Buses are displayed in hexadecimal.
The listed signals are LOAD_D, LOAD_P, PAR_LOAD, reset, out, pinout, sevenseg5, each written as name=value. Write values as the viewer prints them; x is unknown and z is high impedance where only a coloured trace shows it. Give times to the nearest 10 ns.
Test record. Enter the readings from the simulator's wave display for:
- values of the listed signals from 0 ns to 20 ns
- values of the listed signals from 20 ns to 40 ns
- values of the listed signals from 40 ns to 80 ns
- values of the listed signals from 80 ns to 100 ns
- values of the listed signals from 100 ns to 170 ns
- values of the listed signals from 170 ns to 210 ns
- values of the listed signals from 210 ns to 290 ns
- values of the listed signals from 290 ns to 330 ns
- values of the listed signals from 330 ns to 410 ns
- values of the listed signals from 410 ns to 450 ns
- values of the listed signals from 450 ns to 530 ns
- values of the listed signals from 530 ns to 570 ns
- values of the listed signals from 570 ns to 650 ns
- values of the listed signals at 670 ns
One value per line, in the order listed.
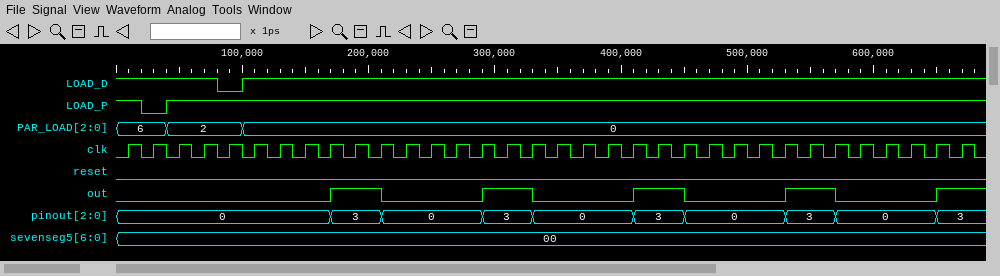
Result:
LOAD_D=1, LOAD_P=1, PAR_LOAD=6, reset=0, out=0, pinout=0, sevenseg5=00
LOAD_D=1, LOAD_P=0, PAR_LOAD=6, reset=0, out=0, pinout=0, sevenseg5=00
LOAD_D=1, LOAD_P=1, PAR_LOAD=2, reset=0, out=0, pinout=0, sevenseg5=00
LOAD_D=0, LOAD_P=1, PAR_LOAD=2, reset=0, out=0, pinout=0, sevenseg5=00
LOAD_D=1, LOAD_P=1, PAR_LOAD=0, reset=0, out=0, pinout=0, sevenseg5=00
LOAD_D=1, LOAD_P=1, PAR_LOAD=0, reset=0, out=1, pinout=3, sevenseg5=00
LOAD_D=1, LOAD_P=1, PAR_LOAD=0, reset=0, out=0, pinout=0, sevenseg5=00
LOAD_D=1, LOAD_P=1, PAR_LOAD=0, reset=0, out=1, pinout=3, sevenseg5=00
LOAD_D=1, LOAD_P=1, PAR_LOAD=0, reset=0, out=0, pinout=0, sevenseg5=00
LOAD_D=1, LOAD_P=1, PAR_LOAD=0, reset=0, out=1, pinout=3, sevenseg5=00
LOAD_D=1, LOAD_P=1, PAR_LOAD=0, reset=0, out=0, pinout=0, sevenseg5=00
LOAD_D=1, LOAD_P=1, PAR_LOAD=0, reset=0, out=1, pinout=3, sevenseg5=00
LOAD_D=1, LOAD_P=1, PAR_LOAD=0, reset=0, out=0, pinout=0, sevenseg5=00
LOAD_D=1, LOAD_P=1, PAR_LOAD=0, reset=0, out=1, pinout=3, sevenseg5=00
